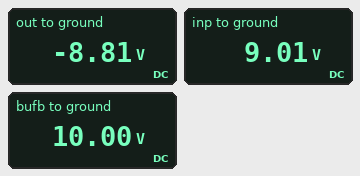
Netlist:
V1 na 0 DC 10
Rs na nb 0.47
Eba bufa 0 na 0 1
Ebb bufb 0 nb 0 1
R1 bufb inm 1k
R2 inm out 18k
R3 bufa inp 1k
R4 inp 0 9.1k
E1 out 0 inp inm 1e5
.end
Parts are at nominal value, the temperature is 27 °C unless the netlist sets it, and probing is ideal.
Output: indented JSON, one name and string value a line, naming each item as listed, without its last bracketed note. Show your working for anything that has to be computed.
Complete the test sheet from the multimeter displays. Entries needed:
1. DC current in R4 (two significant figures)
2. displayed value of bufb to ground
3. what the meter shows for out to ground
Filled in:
{
  "DC current in R4": "(9.01 V) / 9.1 kΩ = 990 µA",
  "displayed value of bufb to ground": "10.00 V",
  "what the meter shows for out to ground": "-8.81 V"
}
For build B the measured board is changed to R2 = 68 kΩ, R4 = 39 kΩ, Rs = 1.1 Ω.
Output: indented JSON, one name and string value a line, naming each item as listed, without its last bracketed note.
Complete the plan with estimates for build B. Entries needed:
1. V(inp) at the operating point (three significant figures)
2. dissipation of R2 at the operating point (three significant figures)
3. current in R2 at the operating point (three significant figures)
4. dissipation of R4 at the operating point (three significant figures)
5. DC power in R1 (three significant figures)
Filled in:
{
  "V(inp) at the operating point": "9.75 V",
  "dissipation of R2 at the operating point": "4.25 mW",
  "current in R2 at the operating point": "250 µA",
  "dissipation of R4 at the operating point": "2.44 mW",
  "DC power in R1": "62.5 µW"
}
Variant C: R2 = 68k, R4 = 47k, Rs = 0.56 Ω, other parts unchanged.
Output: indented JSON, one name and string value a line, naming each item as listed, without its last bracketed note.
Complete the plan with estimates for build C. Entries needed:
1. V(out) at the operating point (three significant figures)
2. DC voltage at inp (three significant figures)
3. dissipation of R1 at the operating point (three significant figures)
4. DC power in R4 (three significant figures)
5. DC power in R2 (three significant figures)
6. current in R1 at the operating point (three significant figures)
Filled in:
{
  "V(out) at the operating point": "-4.37 V",
  "DC voltage at inp": "9.79 V",
  "dissipation of R1 at the operating point": "43.4 µW",
  "DC power in R4": "2.04 mW",
  "DC power in R2": "2.95 mW",
  "current in R1 at the operating point": "208 µA"
}
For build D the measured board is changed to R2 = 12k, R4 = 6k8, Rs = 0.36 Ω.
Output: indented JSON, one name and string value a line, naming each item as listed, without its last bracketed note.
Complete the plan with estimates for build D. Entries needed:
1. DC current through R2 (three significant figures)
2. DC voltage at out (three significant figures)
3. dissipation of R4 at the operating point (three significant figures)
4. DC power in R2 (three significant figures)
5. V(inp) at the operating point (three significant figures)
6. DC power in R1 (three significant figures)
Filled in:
{
  "DC current through R2": "1.28 mA",
  "DC voltage at out": "-6.67 V",
  "dissipation of R4 at the operating point": "11.2 mW",
  "DC power in R2": "19.7 mW",
  "V(inp) at the operating point": "8.72 V",
  "DC power in R1": "1.64 mW"
}
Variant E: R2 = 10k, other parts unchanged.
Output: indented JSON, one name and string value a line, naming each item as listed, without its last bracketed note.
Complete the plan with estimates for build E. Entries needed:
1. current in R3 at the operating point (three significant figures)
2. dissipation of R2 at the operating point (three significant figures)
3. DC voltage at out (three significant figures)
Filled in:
{
  "current in R3 at the operating point": "990 µA",
  "dissipation of R2 at the operating point": "9.80 mW",
  "DC voltage at out": "-891 mV"
}
